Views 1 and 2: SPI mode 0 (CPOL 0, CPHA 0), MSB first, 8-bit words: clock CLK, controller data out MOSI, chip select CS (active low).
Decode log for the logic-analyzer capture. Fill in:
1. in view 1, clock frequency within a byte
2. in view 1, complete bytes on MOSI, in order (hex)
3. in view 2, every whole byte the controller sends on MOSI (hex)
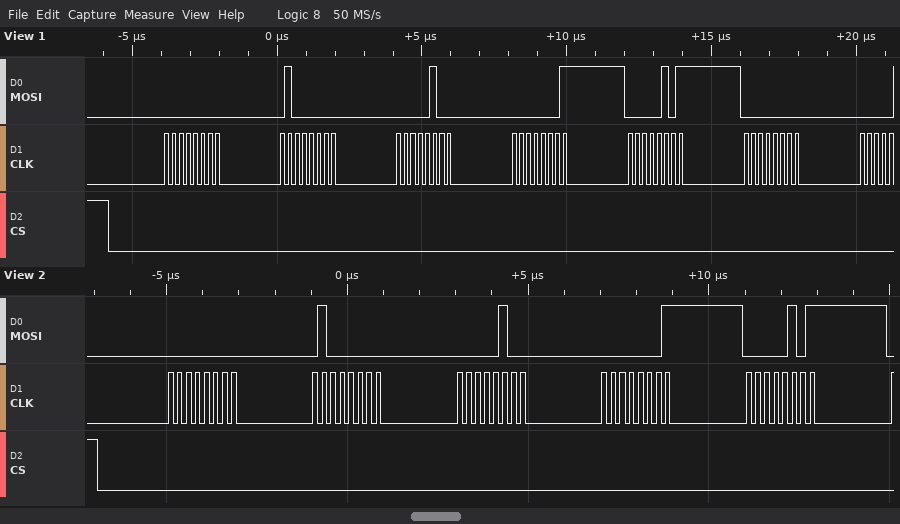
4 MHz
00 40 04 01 05 00
0x00 0x40 0x04 0x01 0x05
